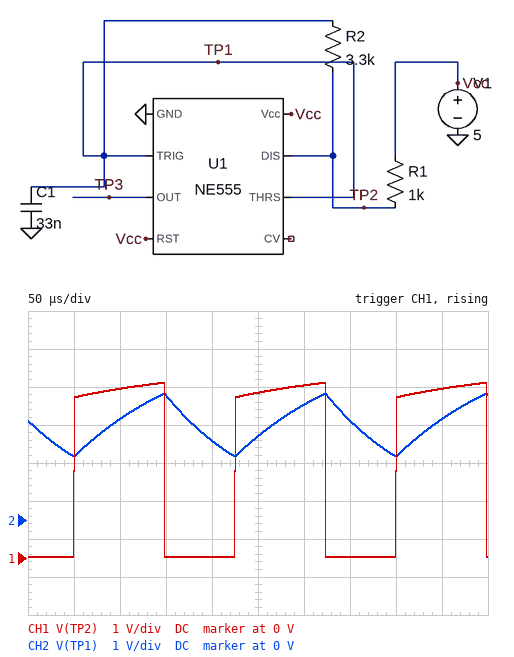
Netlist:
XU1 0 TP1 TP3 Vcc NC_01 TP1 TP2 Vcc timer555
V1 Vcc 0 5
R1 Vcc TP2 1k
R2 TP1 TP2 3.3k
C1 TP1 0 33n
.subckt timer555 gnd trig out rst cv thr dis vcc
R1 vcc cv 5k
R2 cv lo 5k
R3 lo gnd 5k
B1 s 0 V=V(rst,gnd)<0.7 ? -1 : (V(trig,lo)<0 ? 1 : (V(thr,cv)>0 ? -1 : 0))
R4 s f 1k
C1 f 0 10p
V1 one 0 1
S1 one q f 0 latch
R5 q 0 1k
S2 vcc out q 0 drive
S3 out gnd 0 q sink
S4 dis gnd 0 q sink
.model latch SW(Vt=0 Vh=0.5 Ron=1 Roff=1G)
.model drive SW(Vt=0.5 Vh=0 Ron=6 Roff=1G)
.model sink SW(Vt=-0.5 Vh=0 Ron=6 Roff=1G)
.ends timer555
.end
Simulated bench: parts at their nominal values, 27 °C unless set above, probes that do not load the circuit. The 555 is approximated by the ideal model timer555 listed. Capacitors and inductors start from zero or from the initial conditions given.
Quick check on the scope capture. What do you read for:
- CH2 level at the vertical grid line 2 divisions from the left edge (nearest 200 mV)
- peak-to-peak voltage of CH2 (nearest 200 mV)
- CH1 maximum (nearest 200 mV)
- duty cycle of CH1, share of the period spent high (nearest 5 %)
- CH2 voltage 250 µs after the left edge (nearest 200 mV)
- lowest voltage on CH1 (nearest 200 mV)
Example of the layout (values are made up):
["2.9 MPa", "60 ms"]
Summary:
["2.6 V", "1.6 V", "4.6 V", "55 %", "2.2 V", "0 V"]
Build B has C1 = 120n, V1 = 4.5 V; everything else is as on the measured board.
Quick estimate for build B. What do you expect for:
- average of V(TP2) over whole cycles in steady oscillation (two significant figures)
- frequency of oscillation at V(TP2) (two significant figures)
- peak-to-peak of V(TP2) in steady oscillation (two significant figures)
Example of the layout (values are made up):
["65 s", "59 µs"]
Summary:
["2.3 V", "1.6 kHz", "4.1 V"]
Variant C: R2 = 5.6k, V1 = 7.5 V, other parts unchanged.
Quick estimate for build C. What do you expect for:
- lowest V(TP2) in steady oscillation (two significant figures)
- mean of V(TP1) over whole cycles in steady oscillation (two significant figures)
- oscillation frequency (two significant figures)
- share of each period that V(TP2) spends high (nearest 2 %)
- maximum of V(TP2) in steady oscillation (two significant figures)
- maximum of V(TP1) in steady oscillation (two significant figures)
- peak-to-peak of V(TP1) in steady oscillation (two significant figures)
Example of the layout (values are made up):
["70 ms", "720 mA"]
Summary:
["47 mV", "3.8 V", "3.6 kHz", "54 %", "7.1 V", "5.0 V", "2.5 V"]
